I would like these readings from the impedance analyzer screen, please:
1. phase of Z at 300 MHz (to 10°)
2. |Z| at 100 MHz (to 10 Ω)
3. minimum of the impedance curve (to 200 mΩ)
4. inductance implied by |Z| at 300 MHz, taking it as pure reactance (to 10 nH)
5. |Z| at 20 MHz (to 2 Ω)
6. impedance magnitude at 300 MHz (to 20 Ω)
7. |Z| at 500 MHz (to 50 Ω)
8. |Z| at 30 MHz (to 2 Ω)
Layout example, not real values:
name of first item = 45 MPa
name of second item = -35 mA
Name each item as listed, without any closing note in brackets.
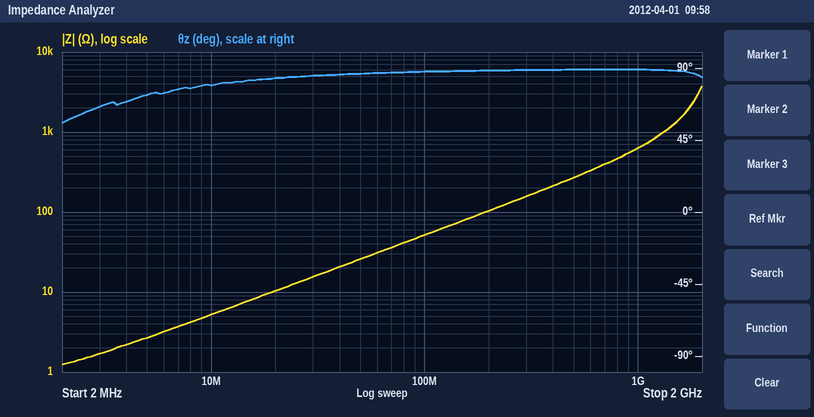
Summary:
phase of Z at 300 MHz = 90°
|Z| at 100 MHz = 50 Ω
minimum of the impedance curve = 1.2 Ω
inductance implied by |Z| at 300 MHz, taking it as pure reactance = 80 nH
|Z| at 20 MHz = 10 Ω
impedance magnitude at 300 MHz = 160 Ω
|Z| at 500 MHz = 250 Ω
|Z| at 30 MHz = 16 Ω
